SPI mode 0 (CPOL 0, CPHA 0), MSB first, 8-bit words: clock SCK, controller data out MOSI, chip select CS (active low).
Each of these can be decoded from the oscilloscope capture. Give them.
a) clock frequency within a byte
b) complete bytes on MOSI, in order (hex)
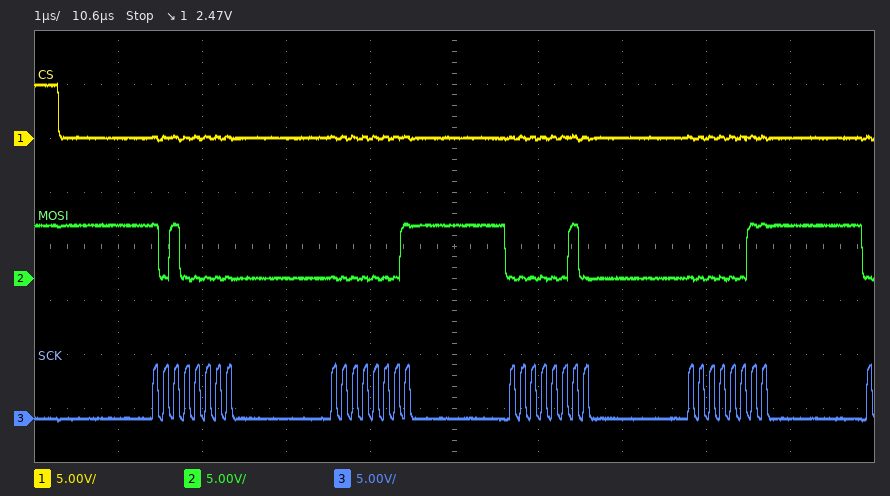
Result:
8 MHz
A0 01 02 03
